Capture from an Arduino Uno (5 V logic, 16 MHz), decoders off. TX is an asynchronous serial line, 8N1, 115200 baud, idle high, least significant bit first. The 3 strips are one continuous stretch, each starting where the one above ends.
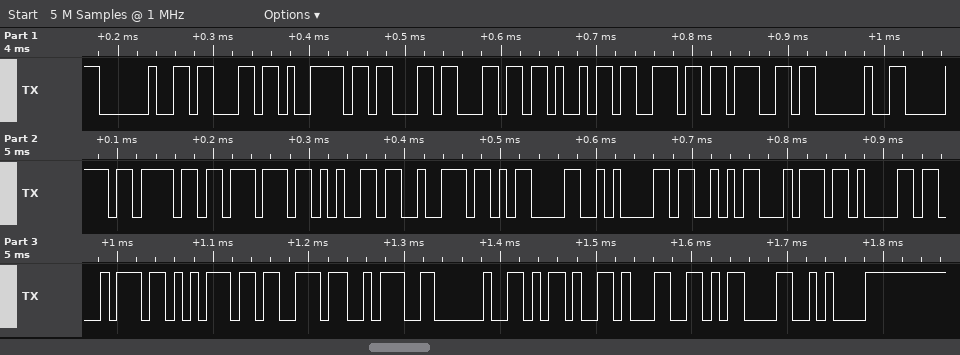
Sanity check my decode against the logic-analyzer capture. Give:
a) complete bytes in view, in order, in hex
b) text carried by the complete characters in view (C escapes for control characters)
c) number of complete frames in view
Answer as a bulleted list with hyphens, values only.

- 20 63 79 63 6C 69 6E 67 20 70 6F 77 65 72 0D 0A 53 74 61 74 75 73 3A 20 2D 31 0D 0A
- " cycling power\r\nStatus: -1\r\n"
- 28
